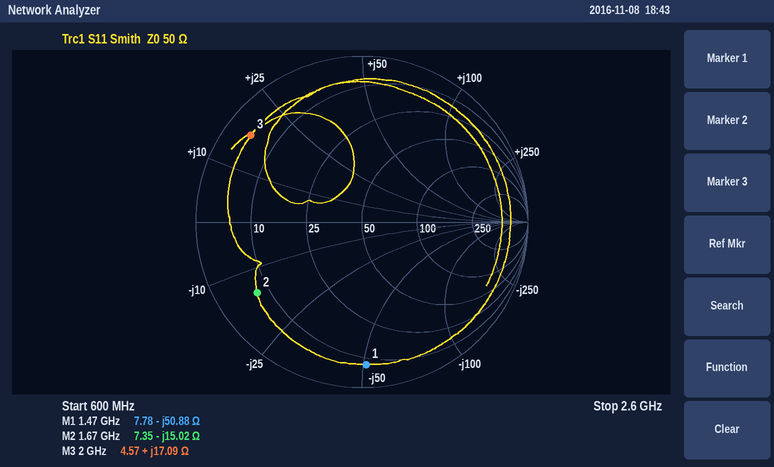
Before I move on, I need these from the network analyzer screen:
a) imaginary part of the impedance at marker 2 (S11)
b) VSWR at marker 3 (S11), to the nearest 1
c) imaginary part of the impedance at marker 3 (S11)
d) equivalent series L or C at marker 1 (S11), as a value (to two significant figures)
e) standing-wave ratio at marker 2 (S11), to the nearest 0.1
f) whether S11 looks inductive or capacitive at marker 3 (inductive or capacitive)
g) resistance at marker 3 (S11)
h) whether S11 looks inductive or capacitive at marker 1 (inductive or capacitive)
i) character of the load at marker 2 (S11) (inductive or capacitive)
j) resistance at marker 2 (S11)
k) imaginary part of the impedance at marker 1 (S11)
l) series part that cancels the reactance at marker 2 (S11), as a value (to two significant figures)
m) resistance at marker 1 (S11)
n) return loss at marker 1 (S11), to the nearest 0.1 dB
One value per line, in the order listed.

-15.02 Ω
12
+17.09 Ω
2.1 pF
7.4
inductive
4.57 Ω
capacitive
capacitive
7.35 Ω
-50.88 Ω
1.4 nH
7.78 Ω
1.3 dB
